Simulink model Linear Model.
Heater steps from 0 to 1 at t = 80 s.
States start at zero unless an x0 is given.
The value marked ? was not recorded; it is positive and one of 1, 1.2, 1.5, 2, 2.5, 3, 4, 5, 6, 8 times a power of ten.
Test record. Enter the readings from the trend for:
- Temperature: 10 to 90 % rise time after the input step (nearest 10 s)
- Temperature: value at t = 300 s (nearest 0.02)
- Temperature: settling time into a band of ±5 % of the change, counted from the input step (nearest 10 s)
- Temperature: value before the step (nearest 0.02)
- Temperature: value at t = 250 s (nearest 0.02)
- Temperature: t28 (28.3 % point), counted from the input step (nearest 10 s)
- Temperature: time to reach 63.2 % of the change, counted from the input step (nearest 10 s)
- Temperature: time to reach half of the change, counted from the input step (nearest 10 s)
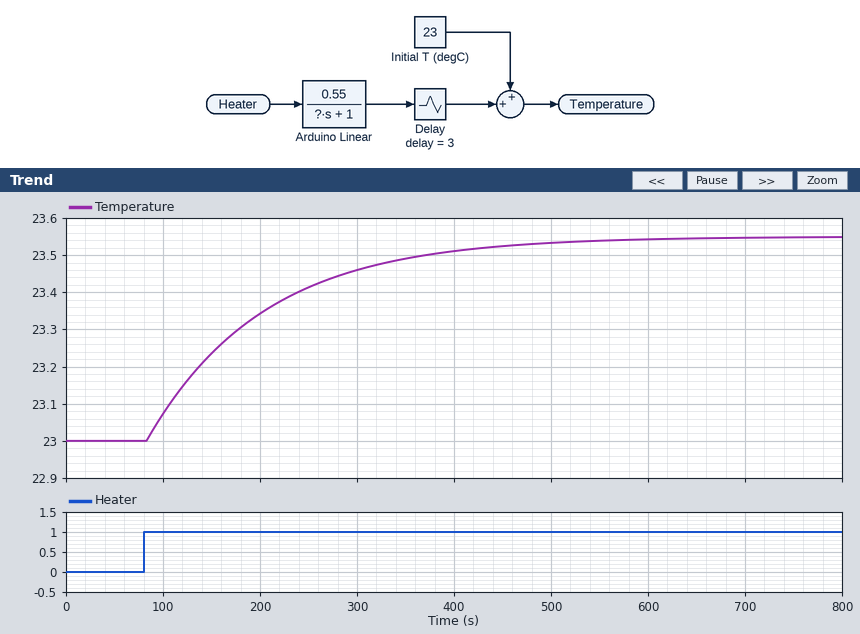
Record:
260 s
23.46
360 s
23.00
23.42
40 s
120 s
90 s
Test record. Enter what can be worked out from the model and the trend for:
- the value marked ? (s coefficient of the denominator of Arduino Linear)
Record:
120
